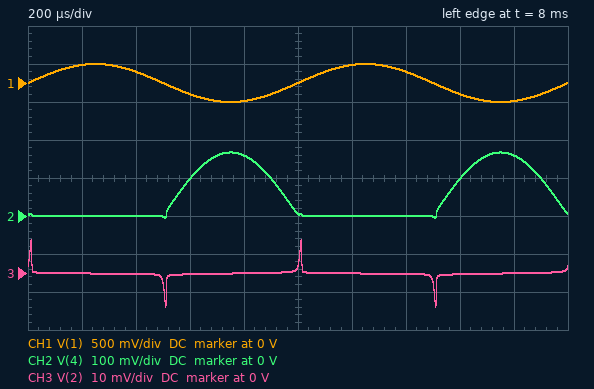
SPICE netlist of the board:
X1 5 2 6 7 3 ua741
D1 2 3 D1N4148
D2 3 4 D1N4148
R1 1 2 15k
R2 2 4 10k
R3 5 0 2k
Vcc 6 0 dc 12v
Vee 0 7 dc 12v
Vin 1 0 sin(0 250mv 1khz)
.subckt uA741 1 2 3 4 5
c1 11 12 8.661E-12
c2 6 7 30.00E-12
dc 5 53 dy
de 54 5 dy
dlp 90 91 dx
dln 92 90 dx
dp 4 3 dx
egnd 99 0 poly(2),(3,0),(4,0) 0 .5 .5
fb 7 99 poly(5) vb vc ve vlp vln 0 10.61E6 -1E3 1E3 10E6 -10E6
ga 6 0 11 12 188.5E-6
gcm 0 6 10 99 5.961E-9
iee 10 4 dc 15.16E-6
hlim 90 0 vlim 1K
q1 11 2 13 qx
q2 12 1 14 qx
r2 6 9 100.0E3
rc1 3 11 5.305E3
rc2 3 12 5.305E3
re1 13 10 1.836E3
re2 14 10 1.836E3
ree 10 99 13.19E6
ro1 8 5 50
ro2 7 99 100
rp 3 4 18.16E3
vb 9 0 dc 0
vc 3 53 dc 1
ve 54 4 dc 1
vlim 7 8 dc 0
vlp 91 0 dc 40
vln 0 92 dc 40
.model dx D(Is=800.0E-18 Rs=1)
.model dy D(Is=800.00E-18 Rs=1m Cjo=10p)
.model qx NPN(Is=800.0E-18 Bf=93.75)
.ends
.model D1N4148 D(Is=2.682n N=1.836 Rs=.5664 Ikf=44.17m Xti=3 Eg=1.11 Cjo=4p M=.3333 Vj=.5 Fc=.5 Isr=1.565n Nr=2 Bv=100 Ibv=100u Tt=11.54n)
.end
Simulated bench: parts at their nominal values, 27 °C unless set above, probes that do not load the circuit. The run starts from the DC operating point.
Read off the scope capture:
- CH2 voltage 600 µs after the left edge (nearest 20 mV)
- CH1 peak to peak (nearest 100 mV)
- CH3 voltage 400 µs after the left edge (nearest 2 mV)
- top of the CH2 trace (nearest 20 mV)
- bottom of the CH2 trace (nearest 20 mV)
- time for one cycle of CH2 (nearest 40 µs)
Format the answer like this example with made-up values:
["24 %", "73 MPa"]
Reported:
["100 mV", "500 mV", "0 V", "160 mV", "0 V", "1.00 ms"]
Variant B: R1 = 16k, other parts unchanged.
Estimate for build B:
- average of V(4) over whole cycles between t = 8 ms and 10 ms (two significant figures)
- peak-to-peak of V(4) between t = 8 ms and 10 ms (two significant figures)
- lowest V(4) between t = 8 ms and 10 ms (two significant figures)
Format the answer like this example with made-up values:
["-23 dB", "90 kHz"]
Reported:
["50 mV", "160 mV", "-5.9 mV"]
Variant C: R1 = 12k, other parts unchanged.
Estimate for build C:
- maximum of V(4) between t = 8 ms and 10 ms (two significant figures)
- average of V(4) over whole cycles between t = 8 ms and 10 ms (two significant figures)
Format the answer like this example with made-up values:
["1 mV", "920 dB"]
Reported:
["210 mV", "66 mV"]
